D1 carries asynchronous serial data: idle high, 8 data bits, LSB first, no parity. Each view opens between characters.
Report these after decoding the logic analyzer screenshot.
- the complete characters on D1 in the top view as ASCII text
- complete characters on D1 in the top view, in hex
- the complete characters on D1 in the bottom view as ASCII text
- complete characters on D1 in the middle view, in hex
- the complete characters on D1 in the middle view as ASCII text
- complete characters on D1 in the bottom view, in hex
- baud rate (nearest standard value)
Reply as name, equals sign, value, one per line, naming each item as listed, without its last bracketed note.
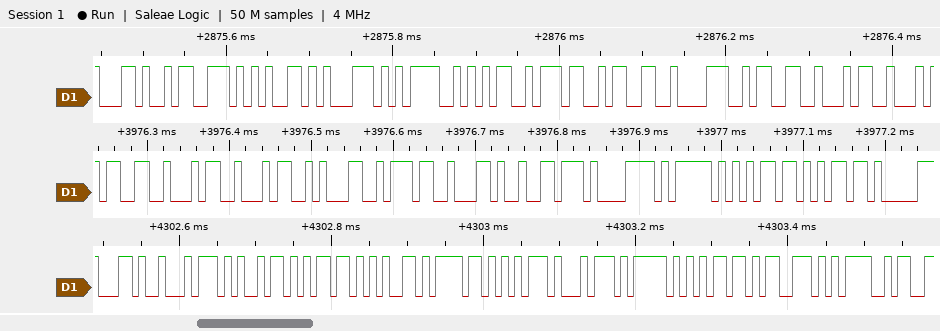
the complete characters on D1 in the top view as ASCII text = ",seq=573834"
complete characters on D1 in the top view, in hex = 2C, 73, 65, 71, 3D, 35, 37, 33, 38, 33, 34
the complete characters on D1 in the bottom view as ASCII text = ",timeout_ms="
complete characters on D1 in the middle view, in hex = 33, 34, 34, 31, 37, 2C, 76, 78, 5F, 6D, 6D
the complete characters on D1 in the middle view as ASCII text = "34417,vx_mm"
complete characters on D1 in the bottom view, in hex = 2C, 74, 69, 6D, 65, 6F, 75, 74, 5F, 6D, 73, 3D
baud rate = 115200 baud
